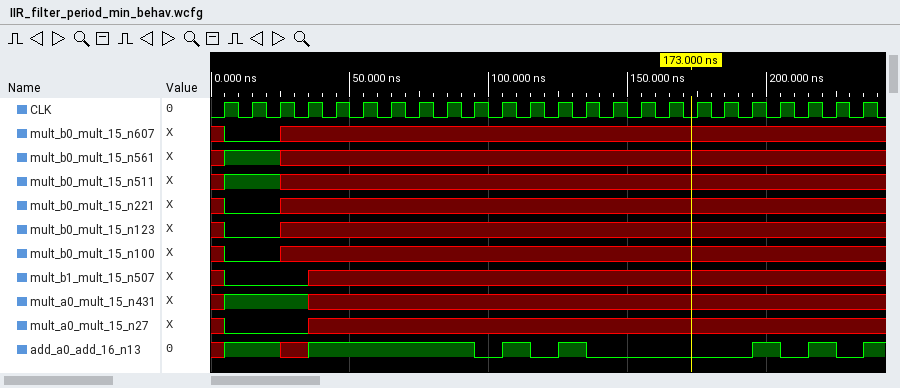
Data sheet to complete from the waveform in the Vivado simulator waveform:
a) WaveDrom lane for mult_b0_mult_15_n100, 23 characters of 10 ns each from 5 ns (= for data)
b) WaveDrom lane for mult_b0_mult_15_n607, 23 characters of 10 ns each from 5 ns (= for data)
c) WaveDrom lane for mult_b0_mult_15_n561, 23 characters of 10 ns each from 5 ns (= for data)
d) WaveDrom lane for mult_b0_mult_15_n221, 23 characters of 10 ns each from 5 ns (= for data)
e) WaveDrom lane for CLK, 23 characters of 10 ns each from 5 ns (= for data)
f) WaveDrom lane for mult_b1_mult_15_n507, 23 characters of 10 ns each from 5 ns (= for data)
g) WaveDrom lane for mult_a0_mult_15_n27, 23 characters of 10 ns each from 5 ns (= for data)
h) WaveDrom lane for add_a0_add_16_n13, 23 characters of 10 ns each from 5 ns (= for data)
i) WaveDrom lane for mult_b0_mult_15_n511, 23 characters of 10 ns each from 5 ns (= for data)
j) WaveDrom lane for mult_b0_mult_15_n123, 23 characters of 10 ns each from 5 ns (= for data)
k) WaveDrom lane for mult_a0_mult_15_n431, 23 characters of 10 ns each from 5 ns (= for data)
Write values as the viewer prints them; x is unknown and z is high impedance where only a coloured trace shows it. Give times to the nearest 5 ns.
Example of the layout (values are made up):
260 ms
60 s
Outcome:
{name: 'mult_b0_mult_15_n100', wave: '0.x....................'}
{name: 'mult_b0_mult_15_n607', wave: '0.x....................'}
{name: 'mult_b0_mult_15_n561', wave: '1.x....................'}
{name: 'mult_b0_mult_15_n221', wave: '0.x....................'}
{name: 'CLK', wave: 'p......................'}
{name: 'mult_b1_mult_15_n507', wave: '0..x...................'}
{name: 'mult_a0_mult_15_n27', wave: '0..x...................'}
{name: 'add_a0_add_16_n13', wave: '1.x1.....01010.....1010'}
{name: 'mult_b0_mult_15_n511', wave: '1.x....................'}
{name: 'mult_b0_mult_15_n123', wave: '0.x....................'}
{name: 'mult_a0_mult_15_n431', wave: '1..x...................'}
